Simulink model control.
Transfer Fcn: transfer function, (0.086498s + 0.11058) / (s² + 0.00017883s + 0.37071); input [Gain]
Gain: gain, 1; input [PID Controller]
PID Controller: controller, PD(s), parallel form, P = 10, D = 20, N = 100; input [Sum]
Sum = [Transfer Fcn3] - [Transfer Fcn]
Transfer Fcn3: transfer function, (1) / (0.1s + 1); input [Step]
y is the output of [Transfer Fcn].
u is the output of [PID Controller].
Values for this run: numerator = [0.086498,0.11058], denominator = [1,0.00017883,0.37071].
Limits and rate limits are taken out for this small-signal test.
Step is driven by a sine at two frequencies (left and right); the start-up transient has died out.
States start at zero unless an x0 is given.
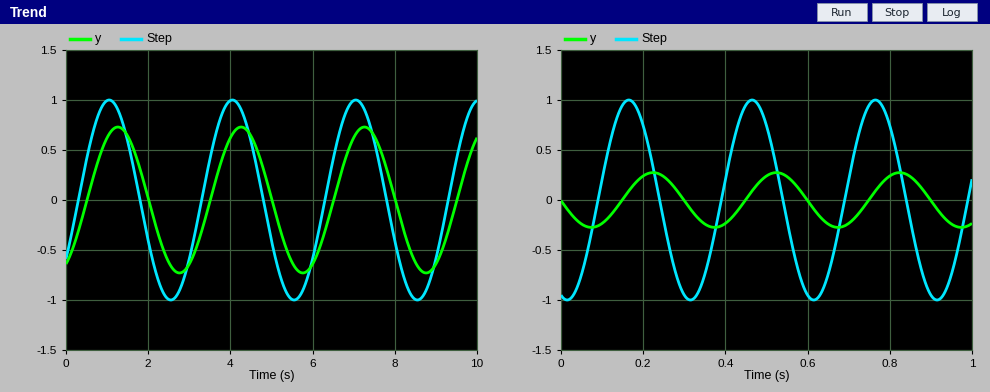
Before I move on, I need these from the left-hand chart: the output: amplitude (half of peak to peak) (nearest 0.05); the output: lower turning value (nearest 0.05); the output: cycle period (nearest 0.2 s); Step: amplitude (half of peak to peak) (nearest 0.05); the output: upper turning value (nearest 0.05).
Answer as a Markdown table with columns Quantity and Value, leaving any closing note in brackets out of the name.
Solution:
| Quantity | Value |
|---|---|
| the output: amplitude (half of peak to peak) | 0.75 |
| the output: lower turning value | -0.75 |
| the output: cycle period | 3.0 s |
| Step: amplitude (half of peak to peak) | 1.00 |
| the output: upper turning value | 0.75 |
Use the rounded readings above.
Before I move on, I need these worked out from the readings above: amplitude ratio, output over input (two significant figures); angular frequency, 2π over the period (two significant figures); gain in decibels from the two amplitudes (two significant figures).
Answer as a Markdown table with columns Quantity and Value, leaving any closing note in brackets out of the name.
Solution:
| Quantity | Value |
|---|---|
| amplitude ratio, output over input | 0.75 |
| angular frequency, 2π over the period | 2.1 rad/s |
| gain in decibels from the two amplitudes | -2.5 dB |
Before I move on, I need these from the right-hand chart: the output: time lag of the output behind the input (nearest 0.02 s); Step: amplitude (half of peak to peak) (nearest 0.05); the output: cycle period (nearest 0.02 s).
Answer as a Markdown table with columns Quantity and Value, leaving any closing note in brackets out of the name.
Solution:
| Quantity | Value |
|---|---|
| the output: time lag of the output behind the input | 0.06 s |
| Step: amplitude (half of peak to peak) | 1.00 |
| the output: cycle period | 0.30 s |
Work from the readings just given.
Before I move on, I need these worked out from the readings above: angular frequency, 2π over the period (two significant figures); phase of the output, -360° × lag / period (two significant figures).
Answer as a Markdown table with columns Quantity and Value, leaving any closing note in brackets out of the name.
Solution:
| Quantity | Value |
|---|---|
| angular frequency, 2π over the period | 21 rad/s |
| phase of the output, -360° × lag / period | -72° |
